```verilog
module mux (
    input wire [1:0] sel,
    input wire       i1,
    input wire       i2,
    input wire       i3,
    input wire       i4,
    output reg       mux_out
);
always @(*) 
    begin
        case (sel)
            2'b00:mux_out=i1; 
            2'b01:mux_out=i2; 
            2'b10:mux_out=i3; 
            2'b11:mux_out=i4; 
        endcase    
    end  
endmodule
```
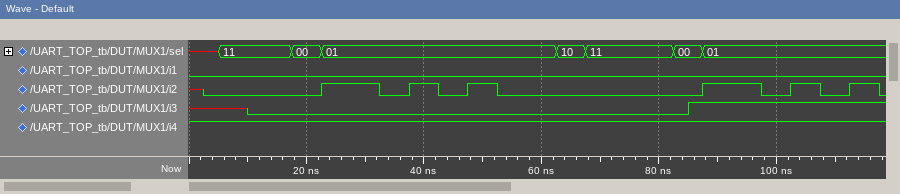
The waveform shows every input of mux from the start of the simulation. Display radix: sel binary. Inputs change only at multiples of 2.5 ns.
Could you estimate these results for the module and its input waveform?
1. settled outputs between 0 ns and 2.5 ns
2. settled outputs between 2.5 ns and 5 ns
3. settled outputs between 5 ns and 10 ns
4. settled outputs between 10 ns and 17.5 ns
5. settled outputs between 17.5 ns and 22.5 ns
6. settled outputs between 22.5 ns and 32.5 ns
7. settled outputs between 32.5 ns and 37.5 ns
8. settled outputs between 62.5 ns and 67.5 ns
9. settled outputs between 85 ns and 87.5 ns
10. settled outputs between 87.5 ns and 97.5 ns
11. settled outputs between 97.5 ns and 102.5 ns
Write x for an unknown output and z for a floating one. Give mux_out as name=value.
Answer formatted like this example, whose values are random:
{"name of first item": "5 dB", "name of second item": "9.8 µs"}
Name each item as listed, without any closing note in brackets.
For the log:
{"settled outputs between 0 ns and 2.5 ns": "mux_out=x", "settled outputs between 2.5 ns and 5 ns": "mux_out=x", "settled outputs between 5 ns and 10 ns": "mux_out=1", "settled outputs between 10 ns and 17.5 ns": "mux_out=1", "settled outputs between 17.5 ns and 22.5 ns": "mux_out=0", "settled outputs between 22.5 ns and 32.5 ns": "mux_out=1", "settled outputs between 32.5 ns and 37.5 ns": "mux_out=0", "settled outputs between 62.5 ns and 67.5 ns": "mux_out=0", "settled outputs between 85 ns and 87.5 ns": "mux_out=0", "settled outputs between 87.5 ns and 97.5 ns": "mux_out=1", "settled outputs between 97.5 ns and 102.5 ns": "mux_out=0"}
